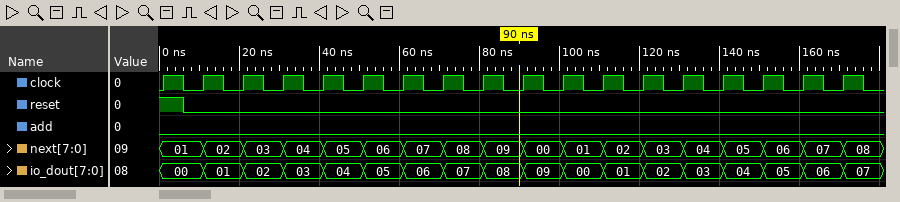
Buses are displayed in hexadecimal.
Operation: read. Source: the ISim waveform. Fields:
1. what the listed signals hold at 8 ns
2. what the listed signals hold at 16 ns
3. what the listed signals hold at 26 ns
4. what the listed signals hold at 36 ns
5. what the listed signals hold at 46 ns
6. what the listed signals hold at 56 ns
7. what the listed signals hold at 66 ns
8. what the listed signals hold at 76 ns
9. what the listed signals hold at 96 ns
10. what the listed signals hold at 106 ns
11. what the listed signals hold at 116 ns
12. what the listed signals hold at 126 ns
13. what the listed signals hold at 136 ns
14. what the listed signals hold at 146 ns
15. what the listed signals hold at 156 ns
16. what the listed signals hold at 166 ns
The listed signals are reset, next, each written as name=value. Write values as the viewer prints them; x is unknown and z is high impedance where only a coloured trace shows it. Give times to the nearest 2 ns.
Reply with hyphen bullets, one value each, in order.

- reset=0, next=01
- reset=0, next=02
- reset=0, next=03
- reset=0, next=04
- reset=0, next=05
- reset=0, next=06
- reset=0, next=07
- reset=0, next=08
- reset=0, next=00
- reset=0, next=01
- reset=0, next=02
- reset=0, next=03
- reset=0, next=04
- reset=0, next=05
- reset=0, next=06
- reset=0, next=07
